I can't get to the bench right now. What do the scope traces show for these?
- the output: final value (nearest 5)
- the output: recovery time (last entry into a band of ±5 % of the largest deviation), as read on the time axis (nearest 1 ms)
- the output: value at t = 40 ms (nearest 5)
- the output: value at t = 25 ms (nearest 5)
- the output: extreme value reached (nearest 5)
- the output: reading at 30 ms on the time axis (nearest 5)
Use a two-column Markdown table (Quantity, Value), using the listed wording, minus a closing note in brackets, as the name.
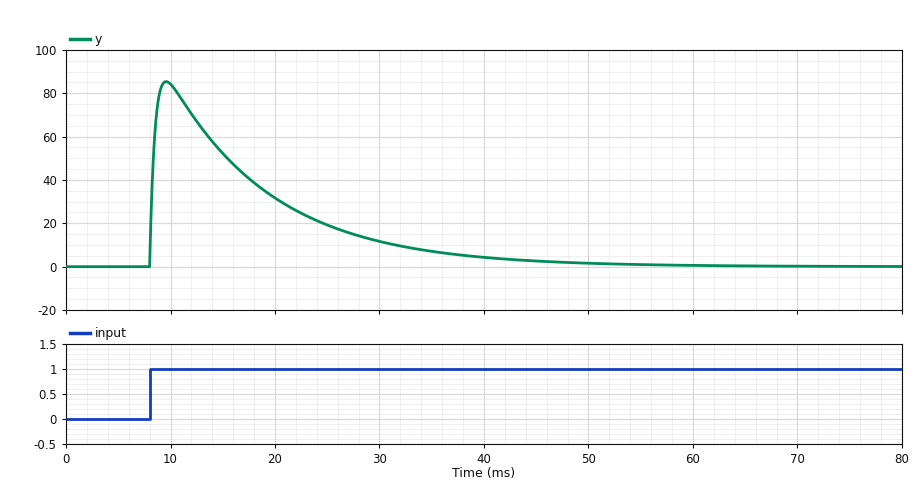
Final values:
| Quantity | Value |
|---|---|
| the output: final value | 0 |
| the output: recovery time (last entry into a band of ±5 % of the largest deviation), as read on the time axis | 40 ms |
| the output: value at t = 40 ms | 5 |
| the output: value at t = 25 ms | 20 |
| the output: extreme value reached | 85 |
| the output: reading at 30 ms on the time axis | 10 |
